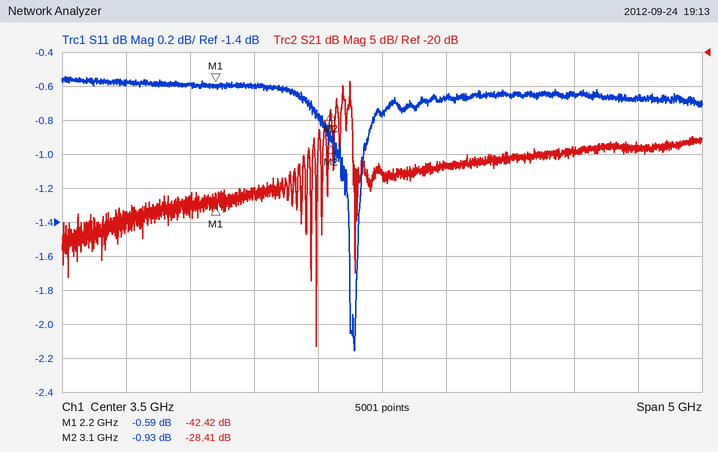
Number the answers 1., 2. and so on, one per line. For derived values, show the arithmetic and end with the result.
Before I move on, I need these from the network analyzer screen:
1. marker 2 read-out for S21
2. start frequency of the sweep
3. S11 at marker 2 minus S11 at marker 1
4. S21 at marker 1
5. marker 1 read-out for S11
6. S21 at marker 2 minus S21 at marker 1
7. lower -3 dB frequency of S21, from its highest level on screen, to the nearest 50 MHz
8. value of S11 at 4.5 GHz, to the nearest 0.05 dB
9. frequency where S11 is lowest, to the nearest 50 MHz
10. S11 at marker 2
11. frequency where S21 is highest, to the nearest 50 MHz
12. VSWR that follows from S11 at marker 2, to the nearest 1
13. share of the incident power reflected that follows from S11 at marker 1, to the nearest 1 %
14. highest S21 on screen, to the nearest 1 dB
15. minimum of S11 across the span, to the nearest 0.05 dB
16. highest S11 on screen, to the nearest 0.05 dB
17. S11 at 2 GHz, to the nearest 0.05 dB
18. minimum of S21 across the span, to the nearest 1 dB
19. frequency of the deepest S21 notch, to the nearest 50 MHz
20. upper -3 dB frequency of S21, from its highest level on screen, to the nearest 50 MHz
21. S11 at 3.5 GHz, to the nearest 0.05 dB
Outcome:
1. -28.41 dB
2. 1 GHz
3. -0.93 − (-0.59) = -0.34 dB
4. -42.42 dB
5. -0.59 dB
6. -28.41 − (-42.42) = 14.01 dB
7. 3.25 GHz
8. -0.65 dB
9. 3.30 GHz
10. -0.93 dB
11. 3.25 GHz
12. (1 + 0.8985)/(1 − 0.8985) ≈ 19
13. 10^(-0.59/10) ≈ 87 %
14. -24 dB
15. -2.15 dB
16. -0.55 dB
17. -0.60 dB
18. -63 dB
19. 3.00 GHz
20. 3.25 GHz
21. -0.75 dB
